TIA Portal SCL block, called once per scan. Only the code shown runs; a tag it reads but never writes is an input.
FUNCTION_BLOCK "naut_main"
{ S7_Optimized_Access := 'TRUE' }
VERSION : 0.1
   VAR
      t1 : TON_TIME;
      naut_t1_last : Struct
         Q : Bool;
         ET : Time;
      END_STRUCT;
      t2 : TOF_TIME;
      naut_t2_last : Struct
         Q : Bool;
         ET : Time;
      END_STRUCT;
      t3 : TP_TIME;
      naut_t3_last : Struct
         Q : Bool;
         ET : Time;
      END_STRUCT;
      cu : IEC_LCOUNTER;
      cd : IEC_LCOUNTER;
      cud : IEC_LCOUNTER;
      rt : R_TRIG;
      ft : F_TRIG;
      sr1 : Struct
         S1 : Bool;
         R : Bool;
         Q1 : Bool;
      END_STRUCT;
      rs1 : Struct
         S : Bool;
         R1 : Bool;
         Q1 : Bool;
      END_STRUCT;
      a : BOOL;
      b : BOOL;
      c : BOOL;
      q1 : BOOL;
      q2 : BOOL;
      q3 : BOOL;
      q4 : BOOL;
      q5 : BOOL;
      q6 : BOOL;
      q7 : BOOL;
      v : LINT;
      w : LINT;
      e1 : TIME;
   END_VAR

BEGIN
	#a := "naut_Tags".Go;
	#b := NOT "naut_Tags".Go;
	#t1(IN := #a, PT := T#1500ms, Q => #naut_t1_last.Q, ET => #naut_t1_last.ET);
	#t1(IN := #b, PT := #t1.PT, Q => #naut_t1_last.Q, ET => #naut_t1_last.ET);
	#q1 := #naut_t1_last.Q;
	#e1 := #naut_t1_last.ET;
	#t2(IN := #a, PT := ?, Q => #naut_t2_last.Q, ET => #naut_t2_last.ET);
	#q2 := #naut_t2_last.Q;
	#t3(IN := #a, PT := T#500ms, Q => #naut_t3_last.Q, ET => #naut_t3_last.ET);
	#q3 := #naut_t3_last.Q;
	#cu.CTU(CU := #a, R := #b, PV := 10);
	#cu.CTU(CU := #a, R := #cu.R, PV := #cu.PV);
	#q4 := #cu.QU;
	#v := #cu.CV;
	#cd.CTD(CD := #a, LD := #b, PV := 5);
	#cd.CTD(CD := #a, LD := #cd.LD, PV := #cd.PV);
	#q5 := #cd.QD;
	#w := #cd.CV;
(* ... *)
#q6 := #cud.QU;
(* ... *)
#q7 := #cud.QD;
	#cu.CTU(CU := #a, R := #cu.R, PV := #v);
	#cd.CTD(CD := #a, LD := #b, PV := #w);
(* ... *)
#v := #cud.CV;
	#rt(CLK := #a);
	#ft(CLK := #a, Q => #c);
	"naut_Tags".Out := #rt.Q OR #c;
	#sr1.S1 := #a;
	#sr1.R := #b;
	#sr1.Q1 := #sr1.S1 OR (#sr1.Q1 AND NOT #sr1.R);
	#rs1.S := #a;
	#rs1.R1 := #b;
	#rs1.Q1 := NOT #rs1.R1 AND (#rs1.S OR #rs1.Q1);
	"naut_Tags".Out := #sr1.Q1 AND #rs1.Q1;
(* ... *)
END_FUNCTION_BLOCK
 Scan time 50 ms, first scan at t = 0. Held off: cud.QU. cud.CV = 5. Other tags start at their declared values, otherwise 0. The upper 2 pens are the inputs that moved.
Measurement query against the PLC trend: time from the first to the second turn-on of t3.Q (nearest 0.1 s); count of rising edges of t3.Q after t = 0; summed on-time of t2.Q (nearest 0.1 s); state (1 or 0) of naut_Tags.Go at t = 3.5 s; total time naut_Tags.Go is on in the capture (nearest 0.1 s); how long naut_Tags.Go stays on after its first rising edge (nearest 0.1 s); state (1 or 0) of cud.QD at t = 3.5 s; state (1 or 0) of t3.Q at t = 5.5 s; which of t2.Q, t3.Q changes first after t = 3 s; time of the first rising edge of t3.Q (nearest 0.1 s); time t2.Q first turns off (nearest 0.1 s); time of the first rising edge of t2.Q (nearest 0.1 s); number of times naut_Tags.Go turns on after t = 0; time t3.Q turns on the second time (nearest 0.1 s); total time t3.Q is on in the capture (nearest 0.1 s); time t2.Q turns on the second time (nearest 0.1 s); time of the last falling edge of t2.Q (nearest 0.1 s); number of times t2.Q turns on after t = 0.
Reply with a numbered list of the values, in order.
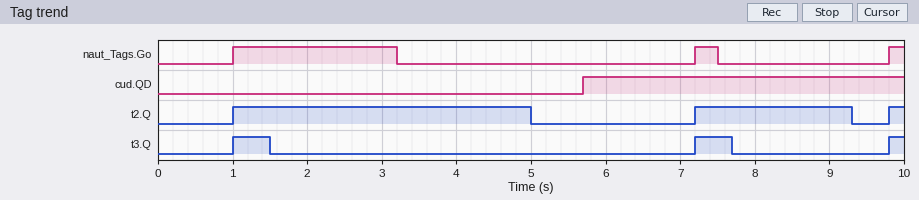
1. 6.2 s
2. 3
3. 6.3 s
4. 0
5. 2.7 s
6. 2.2 s
7. 0
8. 0
9. t2.Q
10. 1.0 s
11. 5.0 s
12. 1.0 s
13. 3
14. 7.2 s
15. 1.2 s
16. 7.2 s
17. 9.3 s
18. 3
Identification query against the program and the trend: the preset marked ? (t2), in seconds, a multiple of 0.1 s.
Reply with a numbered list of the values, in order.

1. 1.8 s
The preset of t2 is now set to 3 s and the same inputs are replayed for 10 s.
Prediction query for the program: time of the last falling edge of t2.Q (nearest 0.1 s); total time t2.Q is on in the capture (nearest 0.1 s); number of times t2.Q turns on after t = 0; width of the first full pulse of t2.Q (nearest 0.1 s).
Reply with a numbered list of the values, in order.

1. 6.2 s
2. 8.0 s
3. 2
4. 5.2 s
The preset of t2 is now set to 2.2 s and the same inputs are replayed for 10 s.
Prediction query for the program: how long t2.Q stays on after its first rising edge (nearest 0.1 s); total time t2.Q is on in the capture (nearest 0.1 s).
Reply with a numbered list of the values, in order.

1. 4.4 s
2. 7.1 s
